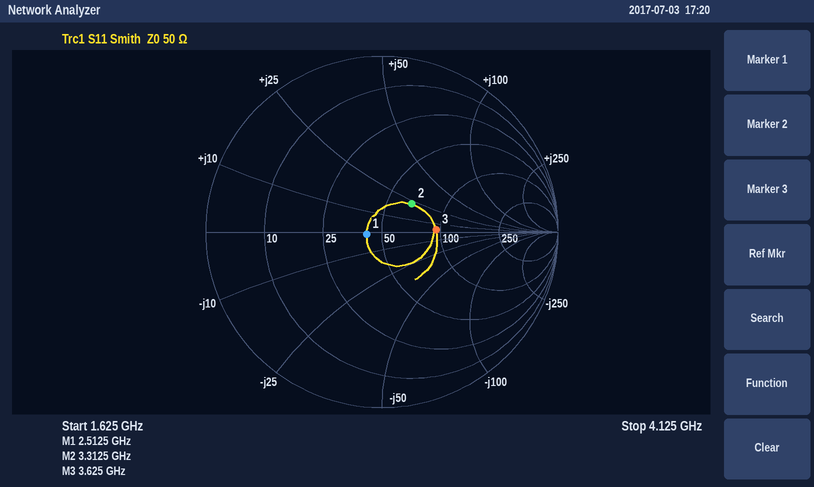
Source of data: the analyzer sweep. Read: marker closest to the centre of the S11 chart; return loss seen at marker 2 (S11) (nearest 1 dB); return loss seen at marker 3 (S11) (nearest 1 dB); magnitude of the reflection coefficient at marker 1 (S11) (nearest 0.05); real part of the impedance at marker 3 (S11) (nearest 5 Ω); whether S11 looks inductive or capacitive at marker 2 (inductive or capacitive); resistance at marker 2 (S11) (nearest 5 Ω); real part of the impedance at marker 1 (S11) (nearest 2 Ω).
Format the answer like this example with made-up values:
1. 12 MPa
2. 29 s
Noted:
1. marker 1
2. 13 dB
3. 10 dB
4. 0.10
5. 95 Ω
6. inductive
7. 65 Ω
8. 42 Ω
